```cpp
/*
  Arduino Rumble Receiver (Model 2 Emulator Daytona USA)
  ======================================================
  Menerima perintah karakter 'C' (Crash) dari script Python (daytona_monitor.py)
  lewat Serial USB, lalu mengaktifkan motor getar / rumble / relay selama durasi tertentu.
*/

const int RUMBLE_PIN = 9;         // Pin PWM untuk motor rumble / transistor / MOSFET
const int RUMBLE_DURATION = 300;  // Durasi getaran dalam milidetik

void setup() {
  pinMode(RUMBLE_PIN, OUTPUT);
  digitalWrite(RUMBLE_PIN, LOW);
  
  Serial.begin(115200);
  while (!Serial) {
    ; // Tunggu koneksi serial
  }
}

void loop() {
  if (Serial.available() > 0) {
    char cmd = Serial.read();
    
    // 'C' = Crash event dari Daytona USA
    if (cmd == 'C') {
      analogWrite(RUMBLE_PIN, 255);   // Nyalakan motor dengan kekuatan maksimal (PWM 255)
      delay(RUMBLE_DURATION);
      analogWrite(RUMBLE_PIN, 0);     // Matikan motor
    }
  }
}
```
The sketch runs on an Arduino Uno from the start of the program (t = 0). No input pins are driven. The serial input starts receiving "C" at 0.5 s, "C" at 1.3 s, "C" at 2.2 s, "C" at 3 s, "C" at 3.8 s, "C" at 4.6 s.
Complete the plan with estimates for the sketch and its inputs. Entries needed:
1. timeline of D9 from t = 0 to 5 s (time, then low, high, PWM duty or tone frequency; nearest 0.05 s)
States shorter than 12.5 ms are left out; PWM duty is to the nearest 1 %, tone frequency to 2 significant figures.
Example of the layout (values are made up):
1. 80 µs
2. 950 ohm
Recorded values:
1. 0 s low; 0.5 s high; 0.8 s low; 1.3 s high; 1.6 s low; 2.2 s high; 2.5 s low; 3 s high; 3.3 s low; 3.8 s high; 4.1 s low; 4.6 s high; 4.9 s low
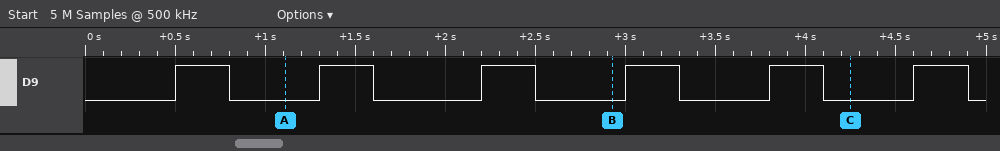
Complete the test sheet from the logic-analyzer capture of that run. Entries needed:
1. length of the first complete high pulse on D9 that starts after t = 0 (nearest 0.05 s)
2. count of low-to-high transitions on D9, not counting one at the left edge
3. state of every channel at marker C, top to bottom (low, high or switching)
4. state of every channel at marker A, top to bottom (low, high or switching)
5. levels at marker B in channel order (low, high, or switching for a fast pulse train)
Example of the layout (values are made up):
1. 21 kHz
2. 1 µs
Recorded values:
1. 0.30 s
2. 6
3. D9 low
4. D9 low
5. D9 low
